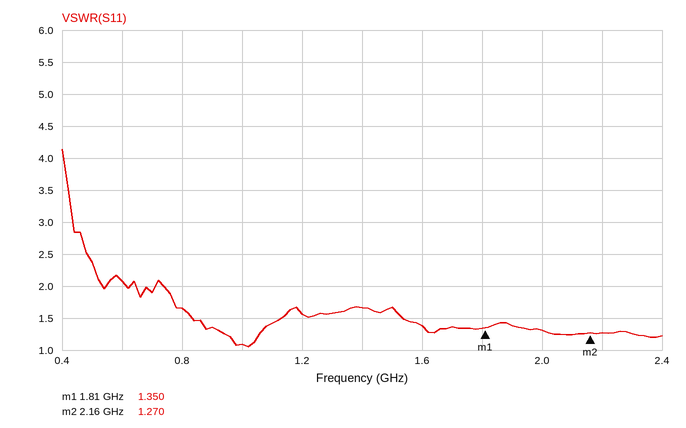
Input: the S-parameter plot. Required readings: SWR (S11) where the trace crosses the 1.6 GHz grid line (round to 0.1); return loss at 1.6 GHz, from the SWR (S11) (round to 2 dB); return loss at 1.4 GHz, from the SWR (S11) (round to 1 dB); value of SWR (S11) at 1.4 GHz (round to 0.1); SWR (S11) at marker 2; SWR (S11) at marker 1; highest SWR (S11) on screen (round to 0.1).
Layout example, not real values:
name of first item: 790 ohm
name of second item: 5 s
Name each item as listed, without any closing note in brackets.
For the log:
SWR (S11) where the trace crosses the 1.6 GHz grid line: 1.4
return loss at 1.6 GHz, from the SWR (S11): 16 dB
return loss at 1.4 GHz, from the SWR (S11): 12 dB
value of SWR (S11) at 1.4 GHz: 1.7
SWR (S11) at marker 2: 1.270
SWR (S11) at marker 1: 1.350
highest SWR (S11) on screen: 4.1
